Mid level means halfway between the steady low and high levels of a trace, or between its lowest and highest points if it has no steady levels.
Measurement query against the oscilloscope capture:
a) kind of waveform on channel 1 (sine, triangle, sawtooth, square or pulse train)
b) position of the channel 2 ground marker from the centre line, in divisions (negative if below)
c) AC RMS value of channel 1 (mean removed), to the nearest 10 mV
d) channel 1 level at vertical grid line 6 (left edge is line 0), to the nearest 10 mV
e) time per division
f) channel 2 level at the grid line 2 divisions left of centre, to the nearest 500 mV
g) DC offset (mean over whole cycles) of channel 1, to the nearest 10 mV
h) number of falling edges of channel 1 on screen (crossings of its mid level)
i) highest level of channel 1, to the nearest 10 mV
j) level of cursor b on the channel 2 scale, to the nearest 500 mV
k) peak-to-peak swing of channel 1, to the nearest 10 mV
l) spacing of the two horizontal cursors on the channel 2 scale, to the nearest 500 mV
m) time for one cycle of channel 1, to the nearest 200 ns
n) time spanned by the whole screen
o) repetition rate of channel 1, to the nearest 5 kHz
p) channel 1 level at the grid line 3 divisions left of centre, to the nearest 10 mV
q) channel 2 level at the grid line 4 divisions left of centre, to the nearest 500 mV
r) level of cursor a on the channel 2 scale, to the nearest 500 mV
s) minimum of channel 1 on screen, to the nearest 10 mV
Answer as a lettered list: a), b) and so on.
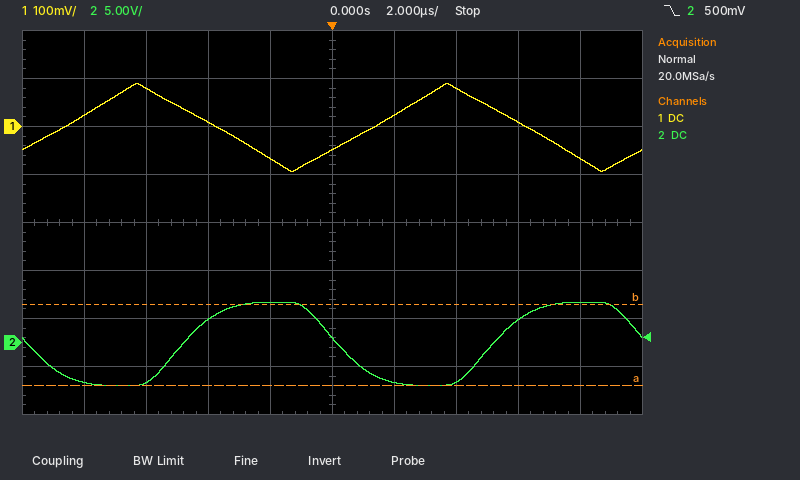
a) triangle
b) -2.5 div
c) 50 mV
d) 20 mV
e) 2 µs
f) 2.5 V
g) 0 mV
h) 2
i) 90 mV
j) 4.0 V
k) 180 mV
l) 8.5 V
m) 10.0 µs
n) 20 µs
o) 100 kHz
p) 80 mV
q) -4.0 V
r) -4.5 V
s) -90 mV
